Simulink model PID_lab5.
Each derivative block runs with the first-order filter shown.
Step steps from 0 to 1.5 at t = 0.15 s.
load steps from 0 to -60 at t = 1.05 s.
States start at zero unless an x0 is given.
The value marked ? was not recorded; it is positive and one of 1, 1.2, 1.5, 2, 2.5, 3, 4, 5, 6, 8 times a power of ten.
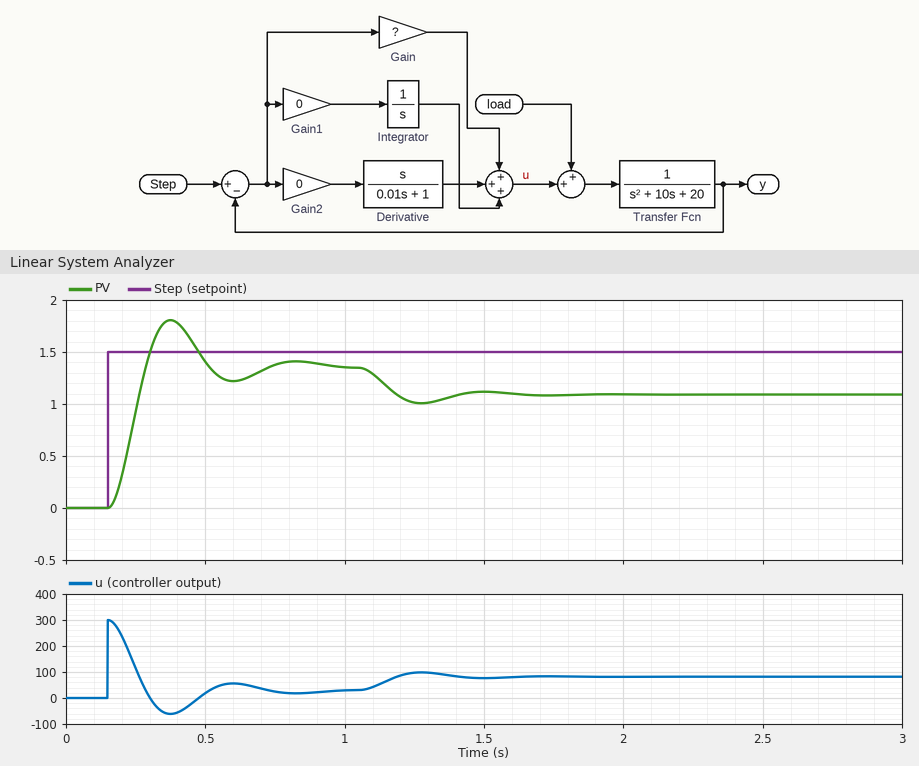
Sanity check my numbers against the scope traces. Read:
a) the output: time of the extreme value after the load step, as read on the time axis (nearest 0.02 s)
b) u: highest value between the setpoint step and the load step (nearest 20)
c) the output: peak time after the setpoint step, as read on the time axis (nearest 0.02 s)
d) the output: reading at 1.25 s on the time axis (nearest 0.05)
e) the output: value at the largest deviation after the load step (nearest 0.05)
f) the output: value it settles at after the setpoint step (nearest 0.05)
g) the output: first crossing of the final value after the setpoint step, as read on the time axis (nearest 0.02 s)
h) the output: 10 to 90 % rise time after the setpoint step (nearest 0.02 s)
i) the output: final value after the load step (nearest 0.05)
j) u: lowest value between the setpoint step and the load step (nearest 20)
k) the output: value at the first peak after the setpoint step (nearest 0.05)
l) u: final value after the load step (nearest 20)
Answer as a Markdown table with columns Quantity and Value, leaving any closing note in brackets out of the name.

| Quantity | Value |
|---|---|
| the output: time of the extreme value after the load step, as read on the time axis | 1.28 s |
| u: highest value between the setpoint step and the load step | 300 |
| the output: peak time after the setpoint step, as read on the time axis | 0.38 s |
| the output: reading at 1.25 s on the time axis | 1.00 |
| the output: value at the largest deviation after the load step | 1.00 |
| the output: value it settles at after the setpoint step | 1.35 |
| the output: first crossing of the final value after the setpoint step, as read on the time axis | 0.28 s |
| the output: 10 to 90 % rise time after the setpoint step | 0.10 s |
| the output: final value after the load step | 1.10 |
| u: lowest value between the setpoint step and the load step | -60 |
| the output: value at the first peak after the setpoint step | 1.80 |
| u: final value after the load step | 80 |
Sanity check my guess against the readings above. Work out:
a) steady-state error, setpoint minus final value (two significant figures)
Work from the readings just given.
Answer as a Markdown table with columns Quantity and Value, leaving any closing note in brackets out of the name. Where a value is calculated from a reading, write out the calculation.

| Quantity | Value |
|---|---|
| steady-state error, setpoint minus final value | 1.5 - 1.35 = 0.15 |
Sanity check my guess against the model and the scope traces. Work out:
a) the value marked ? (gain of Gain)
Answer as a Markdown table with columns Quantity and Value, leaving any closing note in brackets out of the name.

| Quantity | Value |
|---|---|
| the value marked ? | 200 |
